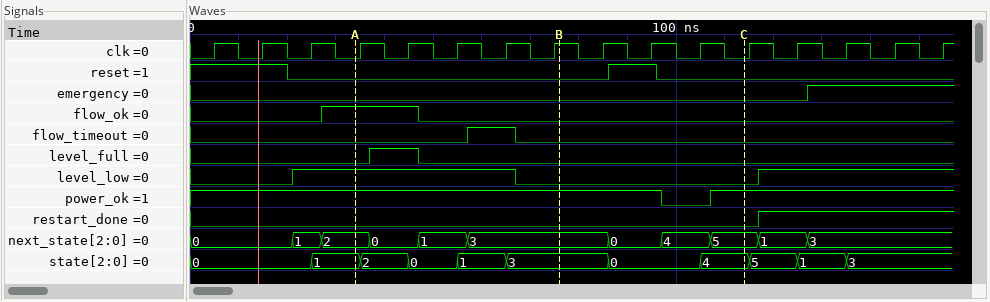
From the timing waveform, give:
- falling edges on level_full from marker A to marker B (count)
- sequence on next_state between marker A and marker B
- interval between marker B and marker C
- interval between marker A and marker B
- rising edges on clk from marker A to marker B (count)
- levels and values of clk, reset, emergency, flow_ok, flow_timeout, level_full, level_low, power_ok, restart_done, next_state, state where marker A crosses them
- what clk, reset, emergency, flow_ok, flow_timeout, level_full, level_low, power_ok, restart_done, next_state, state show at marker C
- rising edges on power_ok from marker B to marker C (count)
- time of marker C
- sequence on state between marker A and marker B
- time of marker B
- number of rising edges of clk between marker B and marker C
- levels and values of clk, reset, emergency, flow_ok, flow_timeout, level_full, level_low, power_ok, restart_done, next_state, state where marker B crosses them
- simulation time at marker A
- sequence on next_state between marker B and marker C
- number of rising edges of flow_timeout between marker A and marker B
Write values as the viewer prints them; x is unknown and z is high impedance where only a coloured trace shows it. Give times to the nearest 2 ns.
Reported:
1
2, 0, 1, 3
38 ns
42 ns
5
clk=0, reset=0, emergency=0, flow_ok=1, flow_timeout=0, level_full=0, level_low=1, power_ok=1, restart_done=0, next_state=2, state=1
clk=0, reset=0, emergency=0, flow_ok=0, flow_timeout=0, level_full=0, level_low=0, power_ok=1, restart_done=0, next_state=5, state=4
1
114 ns
1, 2, 0, 1, 3
76 ns
3
clk=1, reset=0, emergency=0, flow_ok=0, flow_timeout=0, level_full=0, level_low=0, power_ok=1, restart_done=0, next_state=3, state=3
34 ns
3, 0, 4, 5
1
